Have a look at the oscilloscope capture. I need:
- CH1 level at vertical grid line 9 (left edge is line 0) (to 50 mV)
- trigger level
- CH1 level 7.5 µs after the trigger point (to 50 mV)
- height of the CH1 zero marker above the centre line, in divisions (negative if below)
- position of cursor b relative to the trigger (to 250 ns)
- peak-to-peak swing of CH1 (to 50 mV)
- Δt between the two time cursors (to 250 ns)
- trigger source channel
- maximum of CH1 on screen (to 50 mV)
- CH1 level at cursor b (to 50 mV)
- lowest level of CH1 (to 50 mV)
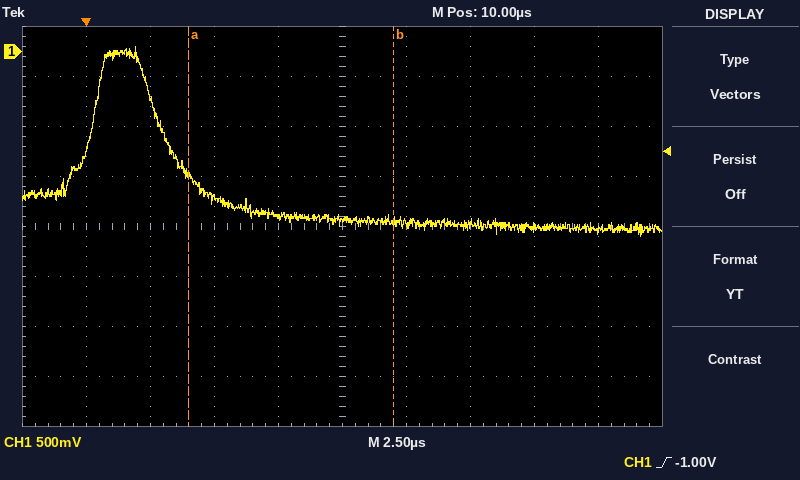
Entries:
-1.80 V
-1.00 V
-1.65 V
+3.5 div
+12.00 µs
1.90 V
8.00 µs
CH1
50 mV
-1.70 V
-1.85 V
